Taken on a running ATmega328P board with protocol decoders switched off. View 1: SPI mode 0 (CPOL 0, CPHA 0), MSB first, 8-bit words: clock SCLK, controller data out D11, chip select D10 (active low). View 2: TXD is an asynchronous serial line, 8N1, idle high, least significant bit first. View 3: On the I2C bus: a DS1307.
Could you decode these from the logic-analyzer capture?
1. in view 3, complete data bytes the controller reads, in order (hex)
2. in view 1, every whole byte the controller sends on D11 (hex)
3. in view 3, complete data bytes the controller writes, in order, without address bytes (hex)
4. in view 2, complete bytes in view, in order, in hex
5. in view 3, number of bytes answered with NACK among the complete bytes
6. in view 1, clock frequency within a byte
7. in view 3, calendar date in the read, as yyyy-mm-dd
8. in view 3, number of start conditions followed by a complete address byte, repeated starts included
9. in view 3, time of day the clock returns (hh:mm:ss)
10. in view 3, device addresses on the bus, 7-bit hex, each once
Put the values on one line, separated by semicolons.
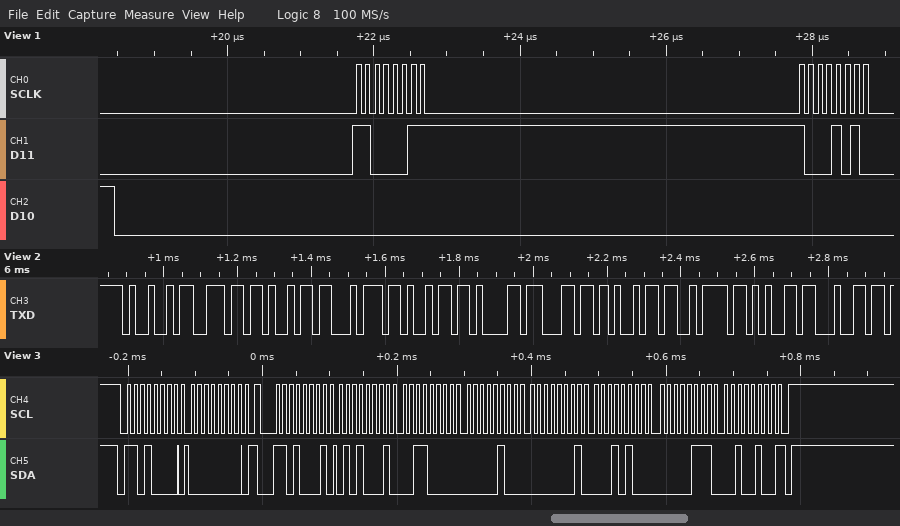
51 30 04 01 14 07 24; C3 8A; 00; 49 6E 69 74 69 61 6C 69 7A 65 64; 1; 8 MHz; 2024-07-14; 2; 04:30:51; 0x68
